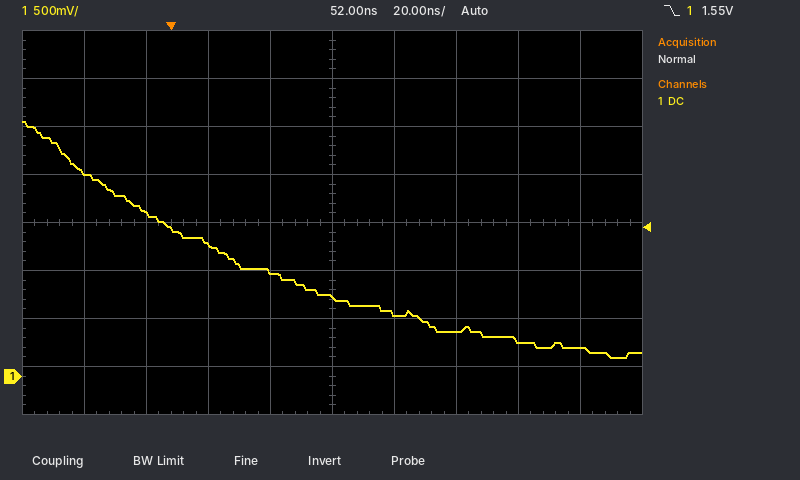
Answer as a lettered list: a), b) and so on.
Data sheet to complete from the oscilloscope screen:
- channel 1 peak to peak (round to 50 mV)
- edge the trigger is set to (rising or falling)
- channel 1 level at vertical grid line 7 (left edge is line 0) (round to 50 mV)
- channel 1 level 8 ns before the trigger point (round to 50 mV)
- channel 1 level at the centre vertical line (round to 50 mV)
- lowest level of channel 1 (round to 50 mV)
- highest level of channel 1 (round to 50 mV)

a) 2.45 V
b) falling
c) 450 mV
d) 1.70 V
e) 800 mV
f) 200 mV
g) 2.65 V
